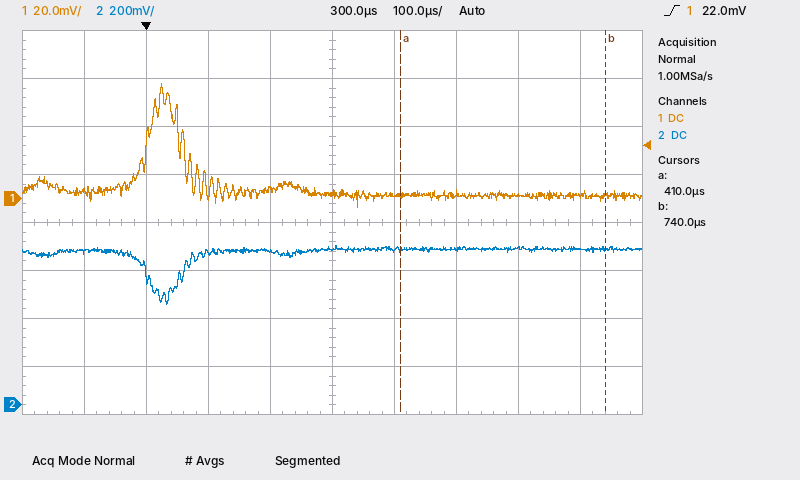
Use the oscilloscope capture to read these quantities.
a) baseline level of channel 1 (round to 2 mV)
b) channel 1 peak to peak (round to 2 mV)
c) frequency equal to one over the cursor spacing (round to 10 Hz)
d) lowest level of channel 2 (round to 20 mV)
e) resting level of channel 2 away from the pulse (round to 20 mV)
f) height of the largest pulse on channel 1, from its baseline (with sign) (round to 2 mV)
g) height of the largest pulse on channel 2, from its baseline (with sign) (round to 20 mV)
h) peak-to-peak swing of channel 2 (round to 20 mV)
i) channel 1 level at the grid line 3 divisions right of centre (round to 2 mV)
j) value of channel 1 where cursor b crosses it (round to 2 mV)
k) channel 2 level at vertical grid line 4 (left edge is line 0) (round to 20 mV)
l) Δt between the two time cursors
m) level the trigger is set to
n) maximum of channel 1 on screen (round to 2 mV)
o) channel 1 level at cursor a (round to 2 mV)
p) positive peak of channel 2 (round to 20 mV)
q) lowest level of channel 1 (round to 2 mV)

2 mV
52 mV
3.03 kHz
420 mV
640 mV
+46 mV
-220 mV
240 mV
2 mV
2 mV
640 mV
330 µs
22.0 mV
48 mV
2 mV
660 mV
-4 mV
